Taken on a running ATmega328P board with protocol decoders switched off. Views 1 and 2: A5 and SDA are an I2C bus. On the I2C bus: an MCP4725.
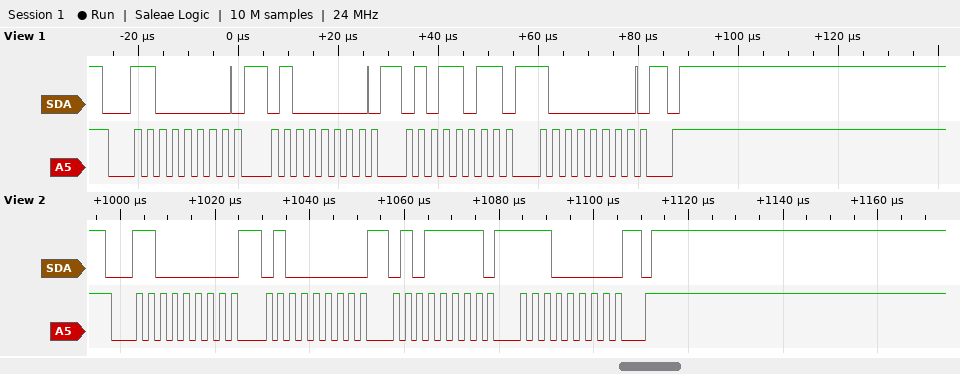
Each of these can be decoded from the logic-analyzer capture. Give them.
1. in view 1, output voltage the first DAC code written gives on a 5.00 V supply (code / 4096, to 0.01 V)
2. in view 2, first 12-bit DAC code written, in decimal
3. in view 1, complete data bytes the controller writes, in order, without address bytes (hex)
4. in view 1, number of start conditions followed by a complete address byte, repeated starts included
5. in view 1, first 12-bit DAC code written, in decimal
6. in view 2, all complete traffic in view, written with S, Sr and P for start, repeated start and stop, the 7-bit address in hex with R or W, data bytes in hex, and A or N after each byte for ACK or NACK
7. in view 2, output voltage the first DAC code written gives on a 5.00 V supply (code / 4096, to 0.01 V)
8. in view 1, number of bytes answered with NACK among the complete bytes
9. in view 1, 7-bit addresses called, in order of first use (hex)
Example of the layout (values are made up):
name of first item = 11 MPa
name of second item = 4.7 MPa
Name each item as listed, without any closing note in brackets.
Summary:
in view 1, output voltage the first DAC code written gives on a 5.00 V supply = 1.79 V
in view 2, first 12-bit DAC code written, in decimal = 1534
in view 1, complete data bytes the controller writes, in order, without address bytes = 40 5B 80
in view 1, number of start conditions followed by a complete address byte, repeated starts included = 1
in view 1, first 12-bit DAC code written, in decimal = 1464
in view 2, all complete traffic in view, written with S, Sr and P for start, repeated start and stop, the 7-bit address in hex with R or W, data bytes in hex, and A or N after each byte for ACK or NACK = S 60W A 40 A 5F A E0 A P
in view 2, output voltage the first DAC code written gives on a 5.00 V supply = 1.87 V
in view 1, number of bytes answered with NACK among the complete bytes = 0
in view 1, 7-bit addresses called, in order of first use = 0x60
